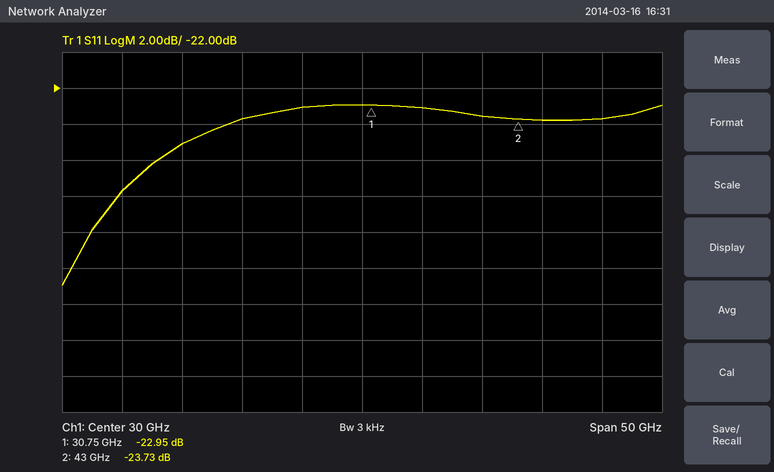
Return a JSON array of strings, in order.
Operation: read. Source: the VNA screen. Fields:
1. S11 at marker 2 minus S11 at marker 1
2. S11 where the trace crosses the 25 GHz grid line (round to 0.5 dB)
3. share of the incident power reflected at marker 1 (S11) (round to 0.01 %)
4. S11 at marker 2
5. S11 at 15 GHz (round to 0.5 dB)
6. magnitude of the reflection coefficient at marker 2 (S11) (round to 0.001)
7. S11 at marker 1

["-0.78 dB", "-23.0 dB", "0.51 %", "-23.73 dB", "-25.0 dB", "0.065", "-22.95 dB"]
